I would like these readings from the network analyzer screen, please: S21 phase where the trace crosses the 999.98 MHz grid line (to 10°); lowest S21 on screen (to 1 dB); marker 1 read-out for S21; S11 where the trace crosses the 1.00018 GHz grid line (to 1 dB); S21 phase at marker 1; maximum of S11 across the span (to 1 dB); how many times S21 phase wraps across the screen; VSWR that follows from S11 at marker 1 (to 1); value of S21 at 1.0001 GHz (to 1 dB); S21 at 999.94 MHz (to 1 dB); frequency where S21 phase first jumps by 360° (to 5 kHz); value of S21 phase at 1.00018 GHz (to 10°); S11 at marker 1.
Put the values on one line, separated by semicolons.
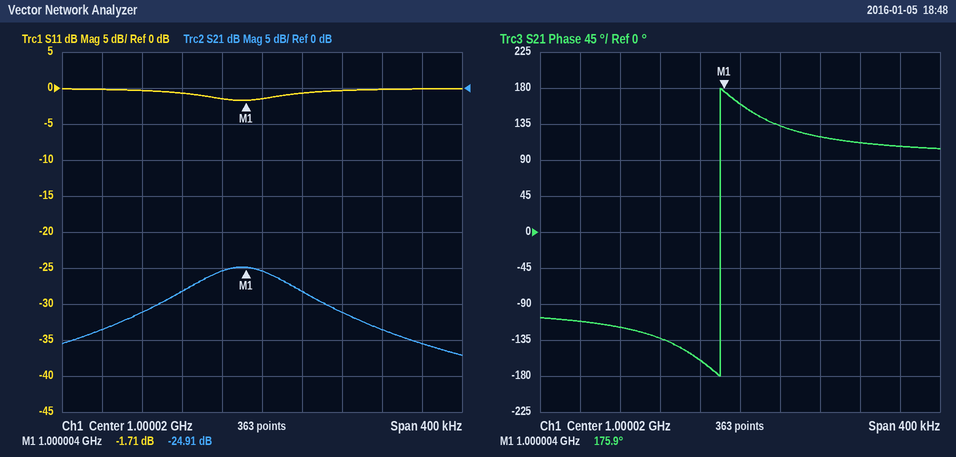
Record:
-160°; -37 dB; -24.91 dB; 0 dB; 175.9°; 0 dB; 1; 10; -31 dB; -28 dB; 1.000000 GHz; 110°; -1.71 dB
